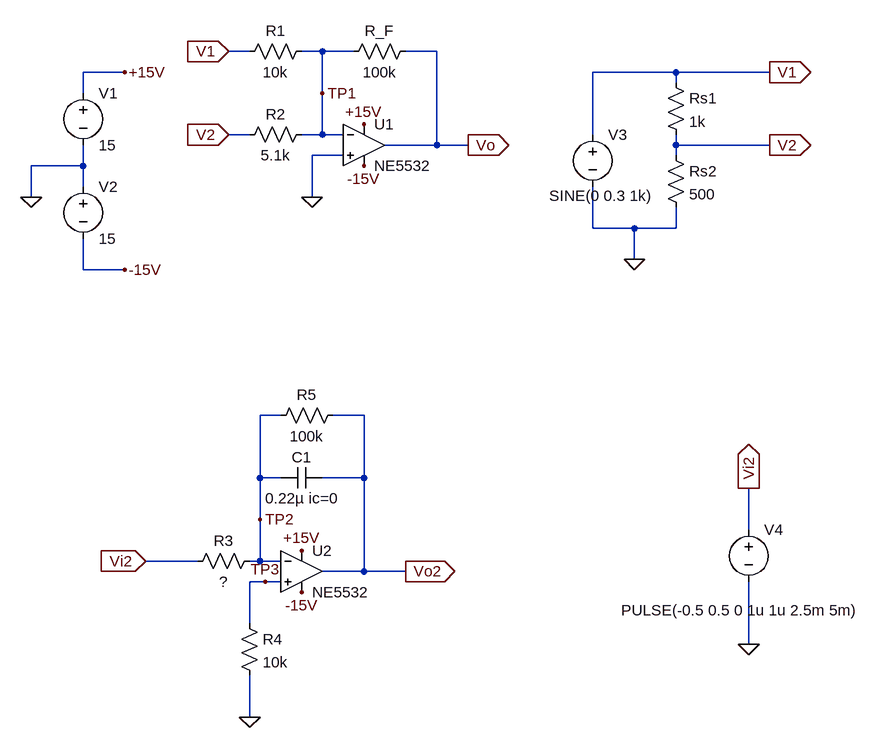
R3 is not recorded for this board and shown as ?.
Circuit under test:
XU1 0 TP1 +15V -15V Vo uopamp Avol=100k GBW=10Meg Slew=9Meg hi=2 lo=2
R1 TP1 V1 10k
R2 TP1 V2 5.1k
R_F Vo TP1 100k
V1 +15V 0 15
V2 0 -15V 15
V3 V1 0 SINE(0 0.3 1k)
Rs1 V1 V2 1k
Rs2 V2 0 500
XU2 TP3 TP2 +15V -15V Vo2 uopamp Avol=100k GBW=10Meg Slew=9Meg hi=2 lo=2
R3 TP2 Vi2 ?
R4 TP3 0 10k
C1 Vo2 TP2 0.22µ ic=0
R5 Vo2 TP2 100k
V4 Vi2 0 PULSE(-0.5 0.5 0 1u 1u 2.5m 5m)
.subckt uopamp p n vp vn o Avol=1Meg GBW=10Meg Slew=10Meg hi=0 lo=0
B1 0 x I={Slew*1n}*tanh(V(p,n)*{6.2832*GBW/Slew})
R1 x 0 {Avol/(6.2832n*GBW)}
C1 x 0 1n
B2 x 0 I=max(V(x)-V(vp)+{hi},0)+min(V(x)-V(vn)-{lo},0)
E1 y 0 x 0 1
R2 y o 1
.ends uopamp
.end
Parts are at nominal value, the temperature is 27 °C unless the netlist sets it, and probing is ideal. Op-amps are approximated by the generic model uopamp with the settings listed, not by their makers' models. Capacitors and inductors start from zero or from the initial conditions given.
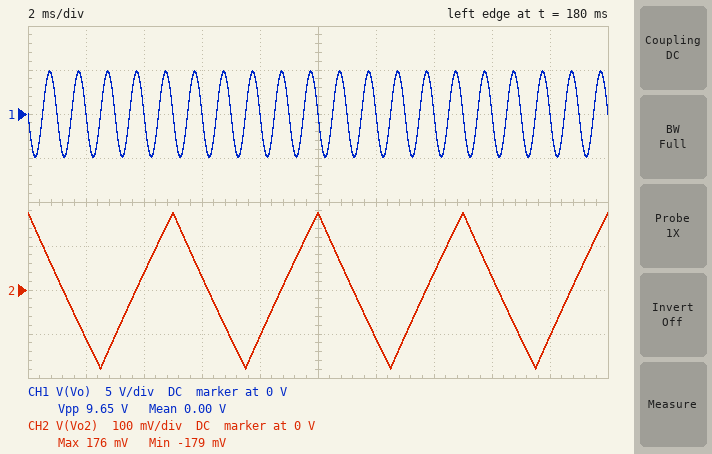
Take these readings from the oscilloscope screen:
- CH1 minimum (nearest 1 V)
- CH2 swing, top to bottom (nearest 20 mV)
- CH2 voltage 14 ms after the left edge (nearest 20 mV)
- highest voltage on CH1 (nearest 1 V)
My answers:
-5 V
360 mV
40 mV
5 V
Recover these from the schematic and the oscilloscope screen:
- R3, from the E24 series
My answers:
16 kΩ
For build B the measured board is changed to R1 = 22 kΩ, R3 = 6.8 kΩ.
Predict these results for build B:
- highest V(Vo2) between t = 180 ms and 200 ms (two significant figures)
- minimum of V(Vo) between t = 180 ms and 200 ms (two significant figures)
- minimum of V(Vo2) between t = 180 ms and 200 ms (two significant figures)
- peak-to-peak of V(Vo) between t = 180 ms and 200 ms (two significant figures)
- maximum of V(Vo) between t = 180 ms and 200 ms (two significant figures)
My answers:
410 mV
-3.2 V
-420 mV
6.4 V
3.2 V
